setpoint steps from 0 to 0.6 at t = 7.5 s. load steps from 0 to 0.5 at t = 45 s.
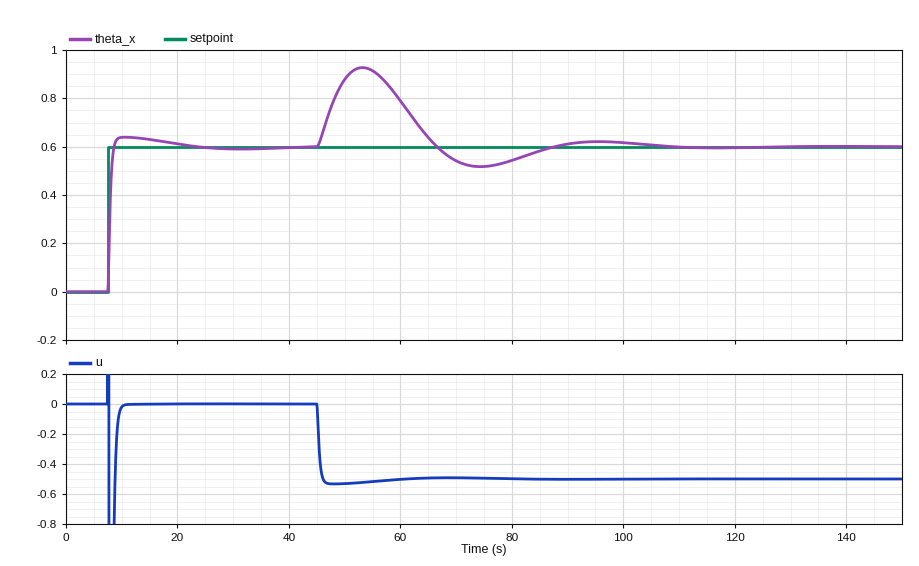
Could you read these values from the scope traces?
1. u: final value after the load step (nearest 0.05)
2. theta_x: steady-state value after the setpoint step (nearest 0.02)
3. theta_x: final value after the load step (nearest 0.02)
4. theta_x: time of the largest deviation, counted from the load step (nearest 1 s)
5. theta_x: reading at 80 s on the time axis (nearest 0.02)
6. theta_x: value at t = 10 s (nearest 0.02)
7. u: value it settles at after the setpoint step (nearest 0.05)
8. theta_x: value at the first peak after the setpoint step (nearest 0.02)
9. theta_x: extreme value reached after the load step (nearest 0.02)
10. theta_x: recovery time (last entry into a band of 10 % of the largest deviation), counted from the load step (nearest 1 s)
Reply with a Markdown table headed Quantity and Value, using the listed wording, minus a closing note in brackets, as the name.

| Quantity | Value |
|---|---|
| u: final value after the load step | -0.50 |
| theta_x: steady-state value after the setpoint step | 0.60 |
| theta_x: final value after the load step | 0.60 |
| theta_x: time of the largest deviation, counted from the load step | 8 s |
| theta_x: reading at 80 s on the time axis | 0.54 |
| theta_x: value at t = 10 s | 0.64 |
| u: value it settles at after the setpoint step | 0.00 |
| theta_x: value at the first peak after the setpoint step | 0.64 |
| theta_x: extreme value reached after the load step | 0.92 |
| theta_x: recovery time (last entry into a band of 10 % of the largest deviation), counted from the load step | 38 s |
